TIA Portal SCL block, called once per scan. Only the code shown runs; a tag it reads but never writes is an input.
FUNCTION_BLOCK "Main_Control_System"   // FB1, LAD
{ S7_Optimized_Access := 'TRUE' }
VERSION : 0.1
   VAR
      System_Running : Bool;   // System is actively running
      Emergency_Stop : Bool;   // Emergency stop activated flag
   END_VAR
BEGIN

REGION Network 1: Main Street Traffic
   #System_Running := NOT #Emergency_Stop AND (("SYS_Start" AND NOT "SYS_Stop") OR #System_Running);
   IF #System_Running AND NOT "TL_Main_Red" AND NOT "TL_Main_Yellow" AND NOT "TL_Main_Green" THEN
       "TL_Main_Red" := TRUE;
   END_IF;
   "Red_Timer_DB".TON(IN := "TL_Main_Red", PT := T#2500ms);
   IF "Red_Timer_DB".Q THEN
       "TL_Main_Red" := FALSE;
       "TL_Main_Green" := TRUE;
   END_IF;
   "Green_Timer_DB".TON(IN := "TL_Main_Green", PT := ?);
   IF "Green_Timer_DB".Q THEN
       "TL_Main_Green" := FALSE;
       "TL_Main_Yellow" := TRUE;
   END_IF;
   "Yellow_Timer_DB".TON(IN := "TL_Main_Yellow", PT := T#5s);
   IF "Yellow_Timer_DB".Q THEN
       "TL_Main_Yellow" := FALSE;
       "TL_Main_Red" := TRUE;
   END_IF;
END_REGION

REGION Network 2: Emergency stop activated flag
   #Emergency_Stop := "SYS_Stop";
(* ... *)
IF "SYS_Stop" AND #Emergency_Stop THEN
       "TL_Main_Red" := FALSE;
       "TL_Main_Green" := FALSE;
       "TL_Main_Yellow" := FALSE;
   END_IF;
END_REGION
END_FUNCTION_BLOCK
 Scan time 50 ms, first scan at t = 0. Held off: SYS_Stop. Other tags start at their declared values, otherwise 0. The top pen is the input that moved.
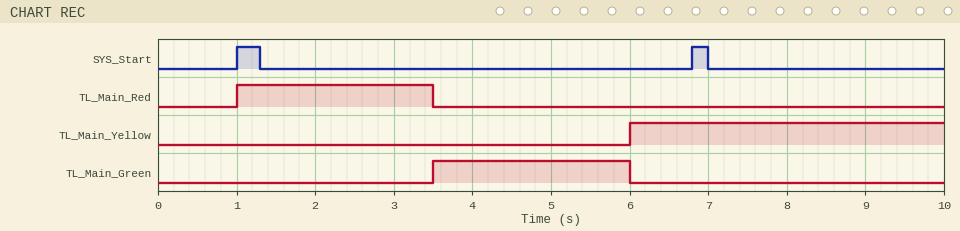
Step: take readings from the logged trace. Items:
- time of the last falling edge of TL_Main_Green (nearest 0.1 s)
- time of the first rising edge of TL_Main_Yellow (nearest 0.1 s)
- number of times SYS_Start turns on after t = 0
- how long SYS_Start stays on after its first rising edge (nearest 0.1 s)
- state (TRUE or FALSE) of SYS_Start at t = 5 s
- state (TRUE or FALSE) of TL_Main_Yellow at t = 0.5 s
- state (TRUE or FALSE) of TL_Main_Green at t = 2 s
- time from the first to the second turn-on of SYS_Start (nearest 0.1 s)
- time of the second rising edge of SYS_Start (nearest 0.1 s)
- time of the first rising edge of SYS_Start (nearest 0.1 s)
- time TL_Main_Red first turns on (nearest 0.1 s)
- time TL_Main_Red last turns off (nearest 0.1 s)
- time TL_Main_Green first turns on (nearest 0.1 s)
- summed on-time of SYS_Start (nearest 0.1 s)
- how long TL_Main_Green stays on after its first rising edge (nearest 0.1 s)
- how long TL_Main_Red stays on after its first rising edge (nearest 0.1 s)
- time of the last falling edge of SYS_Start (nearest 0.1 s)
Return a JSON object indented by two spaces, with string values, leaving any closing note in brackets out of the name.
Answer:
{
  "time of the last falling edge of TL_Main_Green": "6.0 s",
  "time of the first rising edge of TL_Main_Yellow": "6.0 s",
  "number of times SYS_Start turns on after t = 0": "2",
  "how long SYS_Start stays on after its first rising edge": "0.3 s",
  "state (TRUE or FALSE) of SYS_Start at t = 5 s": "FALSE",
  "state (TRUE or FALSE) of TL_Main_Yellow at t = 0.5 s": "FALSE",
  "state (TRUE or FALSE) of TL_Main_Green at t = 2 s": "FALSE",
  "time from the first to the second turn-on of SYS_Start": "5.8 s",
  "time of the second rising edge of SYS_Start": "6.8 s",
  "time of the first rising edge of SYS_Start": "1.0 s",
  "time TL_Main_Red first turns on": "1.0 s",
  "time TL_Main_Red last turns off": "3.5 s",
  "time TL_Main_Green first turns on": "3.5 s",
  "summed on-time of SYS_Start": "0.5 s",
  "how long TL_Main_Green stays on after its first rising edge": "2.5 s",
  "how long TL_Main_Red stays on after its first rising edge": "2.5 s",
  "time of the last falling edge of SYS_Start": "7.0 s"
}
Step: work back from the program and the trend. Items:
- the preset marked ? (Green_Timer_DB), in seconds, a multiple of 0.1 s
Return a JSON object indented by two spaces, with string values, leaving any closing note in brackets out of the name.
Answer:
{
  "the preset marked ? (Green_Timer_DB), in seconds, a multiple of 0.1 s": "2.5 s"
}
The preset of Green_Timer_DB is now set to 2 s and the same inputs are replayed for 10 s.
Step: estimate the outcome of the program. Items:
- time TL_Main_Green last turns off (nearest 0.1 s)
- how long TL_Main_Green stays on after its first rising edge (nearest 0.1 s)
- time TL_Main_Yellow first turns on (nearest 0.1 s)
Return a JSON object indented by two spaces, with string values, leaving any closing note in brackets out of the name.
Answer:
{
  "time TL_Main_Green last turns off": "5.5 s",
  "how long TL_Main_Green stays on after its first rising edge": "2.0 s",
  "time TL_Main_Yellow first turns on": "5.5 s"
}
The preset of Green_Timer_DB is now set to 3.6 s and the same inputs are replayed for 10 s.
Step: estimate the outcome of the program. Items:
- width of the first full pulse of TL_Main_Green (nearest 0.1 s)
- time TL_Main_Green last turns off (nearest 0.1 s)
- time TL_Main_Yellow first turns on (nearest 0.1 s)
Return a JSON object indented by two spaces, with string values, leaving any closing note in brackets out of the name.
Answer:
{
  "width of the first full pulse of TL_Main_Green": "3.6 s",
  "time TL_Main_Green last turns off": "7.1 s",
  "time TL_Main_Yellow first turns on": "7.1 s"
}
